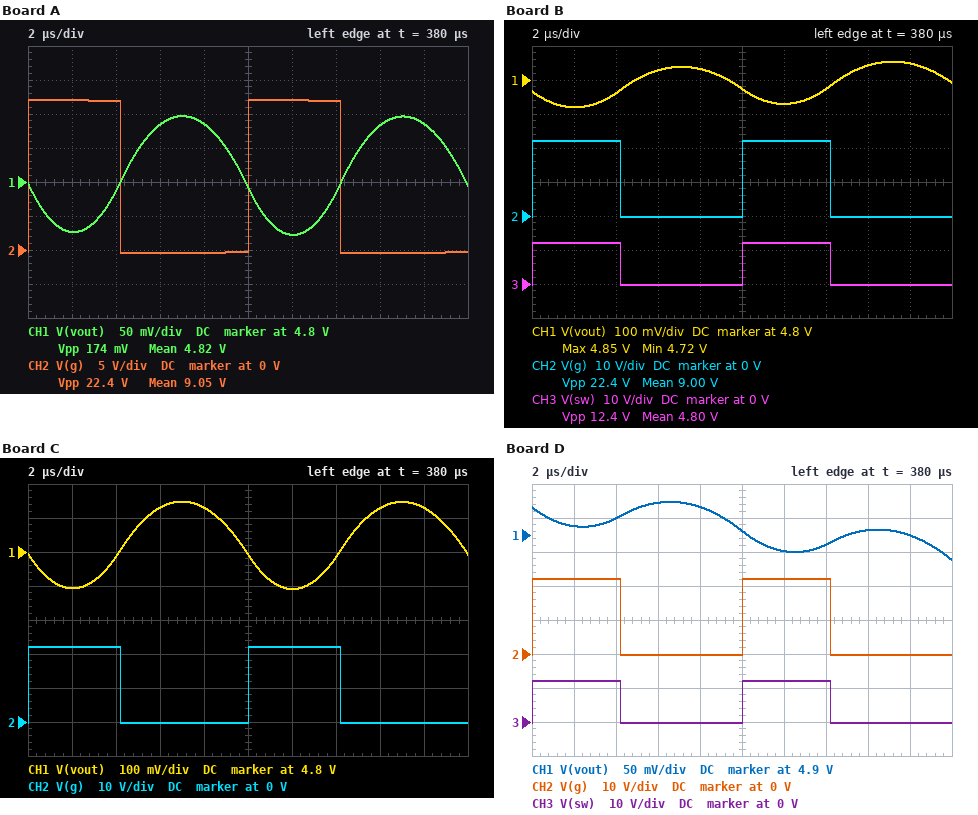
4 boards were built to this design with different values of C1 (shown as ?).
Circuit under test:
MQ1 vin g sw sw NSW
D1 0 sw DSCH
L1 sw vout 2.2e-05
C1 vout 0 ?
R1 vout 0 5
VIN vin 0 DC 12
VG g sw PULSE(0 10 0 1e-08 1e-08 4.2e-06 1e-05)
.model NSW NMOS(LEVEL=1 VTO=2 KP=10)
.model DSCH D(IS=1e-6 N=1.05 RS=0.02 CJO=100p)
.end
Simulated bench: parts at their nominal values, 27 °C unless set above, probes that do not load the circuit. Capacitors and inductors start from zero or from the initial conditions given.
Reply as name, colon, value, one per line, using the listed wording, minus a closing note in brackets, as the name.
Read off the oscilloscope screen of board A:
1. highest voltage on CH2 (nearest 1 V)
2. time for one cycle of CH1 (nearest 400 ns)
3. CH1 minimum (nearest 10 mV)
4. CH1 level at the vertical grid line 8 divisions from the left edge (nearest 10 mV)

highest voltage on CH2: 22 V
time for one cycle of CH1: 10.0 µs
CH1 minimum: 4.72 V
CH1 level at the vertical grid line 8 divisions from the left edge: 4.88 V
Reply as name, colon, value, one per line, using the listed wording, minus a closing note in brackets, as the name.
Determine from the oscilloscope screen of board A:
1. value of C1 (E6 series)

value of C1: 10 µF
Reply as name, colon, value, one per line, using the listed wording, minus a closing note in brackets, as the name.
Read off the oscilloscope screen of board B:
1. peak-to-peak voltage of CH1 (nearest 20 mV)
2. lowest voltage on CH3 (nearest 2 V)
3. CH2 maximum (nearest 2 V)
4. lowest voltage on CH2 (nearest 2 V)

peak-to-peak voltage of CH1: 140 mV
lowest voltage on CH3: 0 V
CH2 maximum: 22 V
lowest voltage on CH2: 0 V
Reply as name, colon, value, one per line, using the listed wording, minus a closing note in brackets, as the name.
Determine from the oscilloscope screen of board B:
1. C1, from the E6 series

C1, from the E6 series: 15 µF
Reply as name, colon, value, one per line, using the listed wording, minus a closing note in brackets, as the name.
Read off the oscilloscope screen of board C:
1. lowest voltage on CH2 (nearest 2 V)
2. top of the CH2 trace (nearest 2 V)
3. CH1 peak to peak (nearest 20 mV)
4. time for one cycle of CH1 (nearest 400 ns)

lowest voltage on CH2: 0 V
top of the CH2 trace: 22 V
CH1 peak to peak: 260 mV
time for one cycle of CH1: 10.0 µs
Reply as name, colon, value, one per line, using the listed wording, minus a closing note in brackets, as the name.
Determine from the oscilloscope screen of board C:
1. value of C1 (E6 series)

value of C1: 6.8 µF
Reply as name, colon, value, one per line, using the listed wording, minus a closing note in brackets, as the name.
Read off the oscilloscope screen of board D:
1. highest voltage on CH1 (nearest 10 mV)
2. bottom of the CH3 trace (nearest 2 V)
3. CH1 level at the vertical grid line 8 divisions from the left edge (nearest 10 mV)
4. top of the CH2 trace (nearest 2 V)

highest voltage on CH1: 4.95 V
bottom of the CH3 trace: 0 V
CH1 level at the vertical grid line 8 divisions from the left edge: 4.91 V
top of the CH2 trace: 22 V
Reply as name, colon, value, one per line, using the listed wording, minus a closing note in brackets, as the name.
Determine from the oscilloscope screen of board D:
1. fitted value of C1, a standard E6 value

fitted value of C1, a standard E6 value: 33 µF
